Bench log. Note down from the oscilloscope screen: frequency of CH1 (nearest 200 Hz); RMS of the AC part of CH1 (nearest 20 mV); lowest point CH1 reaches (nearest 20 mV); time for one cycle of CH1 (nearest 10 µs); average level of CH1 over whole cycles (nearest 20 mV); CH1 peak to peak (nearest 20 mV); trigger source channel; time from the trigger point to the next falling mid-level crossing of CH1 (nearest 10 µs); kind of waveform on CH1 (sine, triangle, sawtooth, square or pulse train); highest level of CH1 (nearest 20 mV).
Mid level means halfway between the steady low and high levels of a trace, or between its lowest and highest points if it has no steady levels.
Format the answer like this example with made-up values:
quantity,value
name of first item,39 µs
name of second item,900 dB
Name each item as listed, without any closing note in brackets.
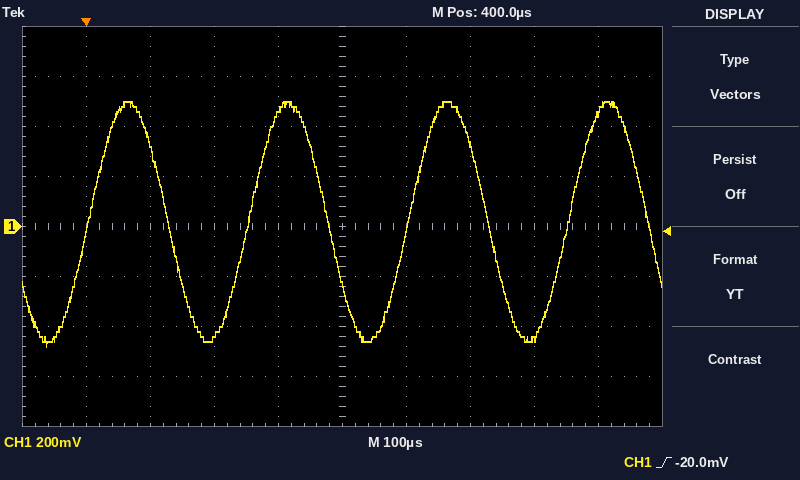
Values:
quantity,value
frequency of CH1,4.0 kHz
RMS of the AC part of CH1,340 mV
lowest point CH1 reaches,-480 mV
time for one cycle of CH1,250 µs
average level of CH1 over whole cycles,20 mV
CH1 peak to peak,980 mV
trigger source channel,CH1
time from the trigger point to the next falling mid-level crossing of CH1,130 µs
kind of waveform on CH1,sine
highest level of CH1,500 mV
